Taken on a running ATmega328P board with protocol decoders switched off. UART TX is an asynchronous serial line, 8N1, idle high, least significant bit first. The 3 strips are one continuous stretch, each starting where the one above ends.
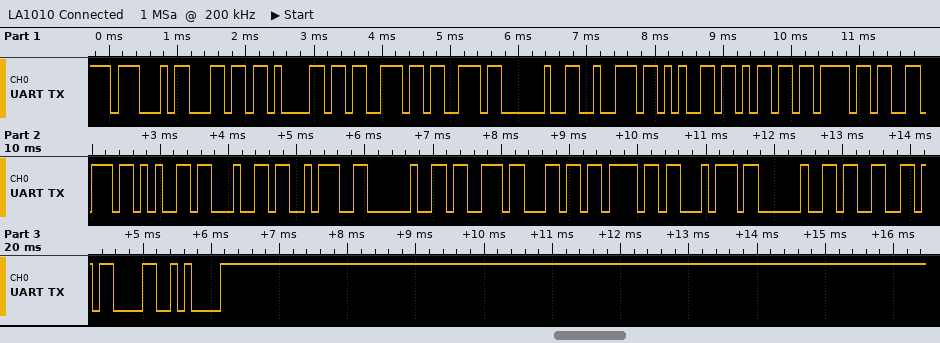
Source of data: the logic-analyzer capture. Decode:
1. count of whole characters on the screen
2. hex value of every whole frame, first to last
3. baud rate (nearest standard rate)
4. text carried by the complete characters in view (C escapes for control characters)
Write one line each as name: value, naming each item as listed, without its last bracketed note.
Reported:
count of whole characters on the screen: 23
hex value of every whole frame, first to last: 47 6C 61 73 73 20 72 65 6D 6F 76 65 64 3A 20 73 6C 6F 74 20 33 0D 0A
baud rate: 9600 baud
text carried by the complete characters in view: "Glass removed: slot 3\r\n"
